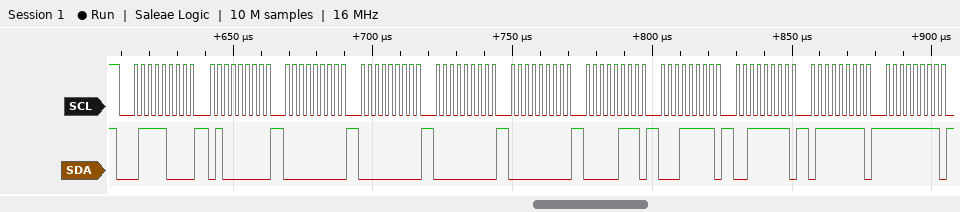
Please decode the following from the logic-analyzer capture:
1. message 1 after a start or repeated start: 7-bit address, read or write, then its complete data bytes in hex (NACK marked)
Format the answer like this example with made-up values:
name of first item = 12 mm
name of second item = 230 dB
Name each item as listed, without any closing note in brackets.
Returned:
message 1 after a start or repeated start: 7-bit address, read or write, then its complete data bytes in hex = 0x3C write: 40 00 00 00 00 07 1F 3F 7F FF
